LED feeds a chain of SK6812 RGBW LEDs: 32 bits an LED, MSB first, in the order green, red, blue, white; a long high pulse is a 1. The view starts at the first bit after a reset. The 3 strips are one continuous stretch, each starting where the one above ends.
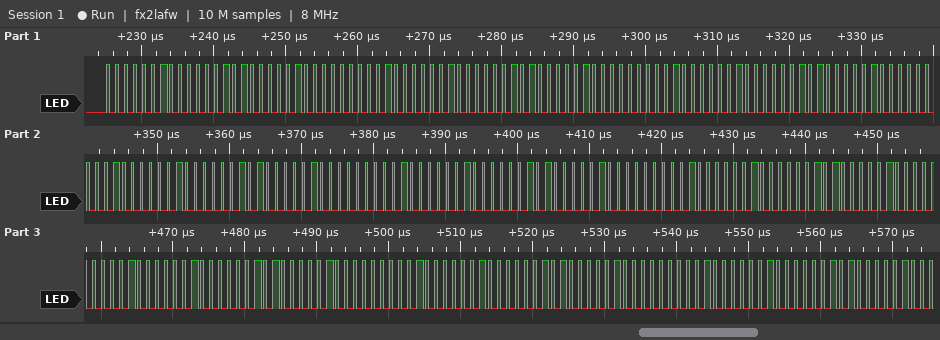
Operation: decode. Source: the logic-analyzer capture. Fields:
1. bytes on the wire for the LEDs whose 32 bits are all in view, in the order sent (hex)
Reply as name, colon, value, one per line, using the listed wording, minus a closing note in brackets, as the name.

bytes on the wire for the LEDs whose 32 bits are all in view, in the order sent: 02 05 04 01 02 05 04 01 02 05 04 01 02 05 04 01 02 05 04 01 02 05 04 01 02 05 04 01 02 05 04 01
